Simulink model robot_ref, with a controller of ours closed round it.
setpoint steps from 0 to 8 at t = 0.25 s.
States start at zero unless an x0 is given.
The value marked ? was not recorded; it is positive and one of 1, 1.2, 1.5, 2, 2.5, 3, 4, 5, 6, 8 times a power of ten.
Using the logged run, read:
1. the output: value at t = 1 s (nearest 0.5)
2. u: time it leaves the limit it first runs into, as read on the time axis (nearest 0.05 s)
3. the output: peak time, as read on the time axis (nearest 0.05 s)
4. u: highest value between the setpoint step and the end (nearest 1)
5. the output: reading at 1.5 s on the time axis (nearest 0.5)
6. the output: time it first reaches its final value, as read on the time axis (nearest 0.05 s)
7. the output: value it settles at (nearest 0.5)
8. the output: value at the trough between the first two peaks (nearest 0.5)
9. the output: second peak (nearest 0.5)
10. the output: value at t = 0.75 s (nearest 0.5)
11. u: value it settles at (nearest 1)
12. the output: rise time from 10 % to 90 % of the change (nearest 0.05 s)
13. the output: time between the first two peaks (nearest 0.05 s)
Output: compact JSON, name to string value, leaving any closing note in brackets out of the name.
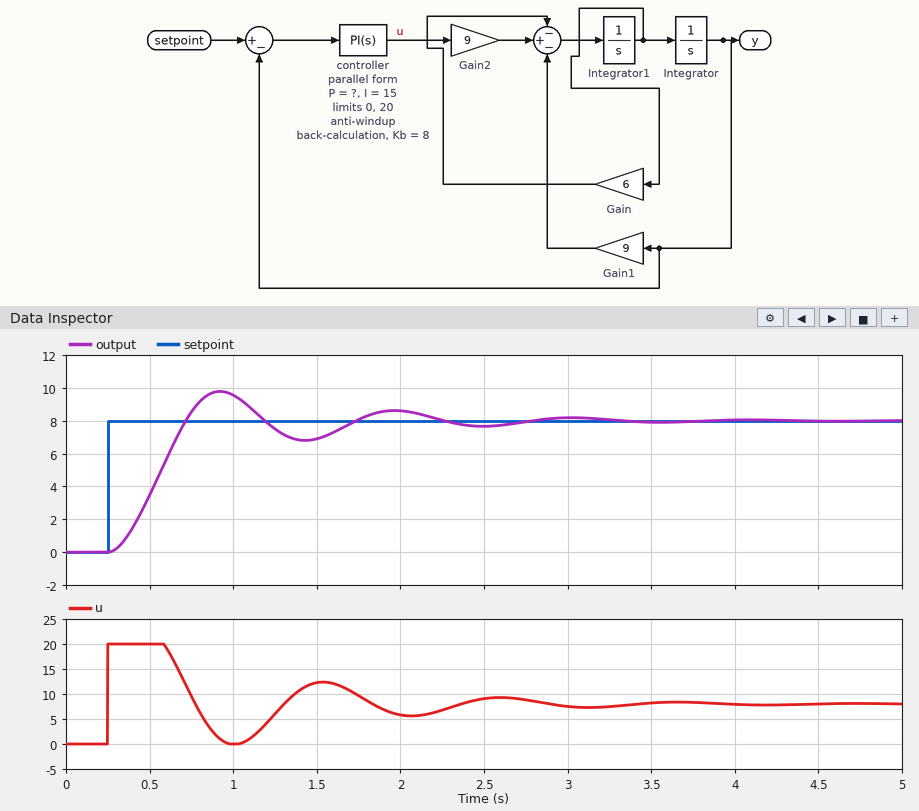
{"the output: value at t = 1 s": "9.5", "u: time it leaves the limit it first runs into, as read on the time axis": "0.60 s", "the output: peak time, as read on the time axis": "0.90 s", "u: highest value between the setpoint step and the end": "20", "the output: reading at 1.5 s on the time axis": "7.0", "the output: time it first reaches its final value, as read on the time axis": "0.70 s", "the output: value it settles at": "8.0", "the output: value at the trough between the first two peaks": "7.0", "the output: second peak": "8.5", "the output: value at t = 0.75 s": "8.5", "u: value it settles at": "8", "the output: rise time from 10 % to 90 % of the change": "0.30 s", "the output: time between the first two peaks": "1.05 s"}
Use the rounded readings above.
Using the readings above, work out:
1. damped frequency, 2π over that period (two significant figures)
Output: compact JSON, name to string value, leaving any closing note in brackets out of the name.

{"damped frequency, 2π over that period": "6.0 rad/s"}
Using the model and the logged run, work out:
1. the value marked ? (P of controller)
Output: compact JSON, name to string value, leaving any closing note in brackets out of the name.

{"the value marked ?": "4"}
